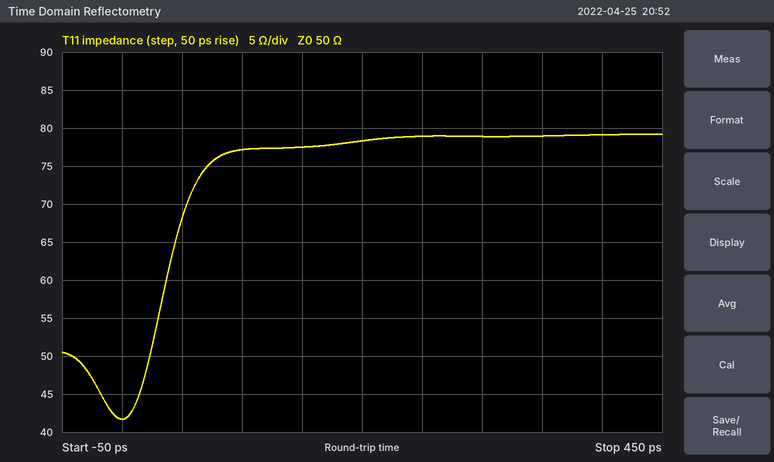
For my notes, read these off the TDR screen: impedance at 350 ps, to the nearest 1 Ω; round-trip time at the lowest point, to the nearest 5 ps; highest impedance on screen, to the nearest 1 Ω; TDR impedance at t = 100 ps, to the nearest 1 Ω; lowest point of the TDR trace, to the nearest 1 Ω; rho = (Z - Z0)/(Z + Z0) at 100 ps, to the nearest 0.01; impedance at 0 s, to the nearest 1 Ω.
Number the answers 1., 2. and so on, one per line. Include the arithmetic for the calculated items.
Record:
1. 79 Ω
2. 0 ps
3. 79 Ω
4. 77 Ω
5. 42 Ω
6. (77 − 50)/(77 + 50) ≈ +0.21
7. 42 Ω
